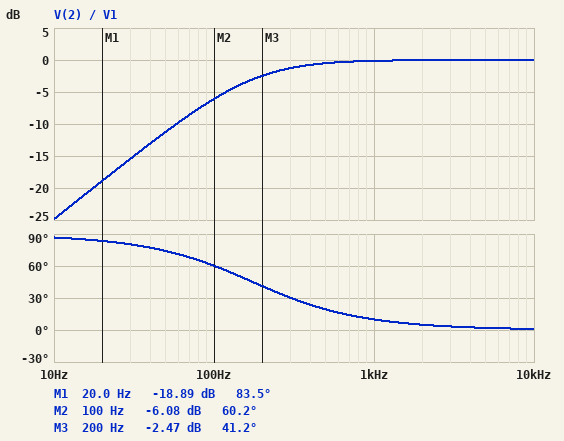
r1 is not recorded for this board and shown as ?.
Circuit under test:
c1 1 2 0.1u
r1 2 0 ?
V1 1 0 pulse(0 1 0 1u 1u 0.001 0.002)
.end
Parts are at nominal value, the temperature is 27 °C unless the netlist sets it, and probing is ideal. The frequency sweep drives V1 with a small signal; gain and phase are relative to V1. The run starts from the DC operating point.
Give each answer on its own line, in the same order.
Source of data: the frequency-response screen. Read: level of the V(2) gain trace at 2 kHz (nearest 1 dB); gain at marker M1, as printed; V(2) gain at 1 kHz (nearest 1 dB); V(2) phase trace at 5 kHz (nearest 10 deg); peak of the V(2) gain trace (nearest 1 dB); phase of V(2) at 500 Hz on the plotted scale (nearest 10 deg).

0 dB
-18.89 dB
0 dB
0 deg
0 dB
20 deg
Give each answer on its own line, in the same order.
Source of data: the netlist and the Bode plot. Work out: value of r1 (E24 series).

9.1 kΩ
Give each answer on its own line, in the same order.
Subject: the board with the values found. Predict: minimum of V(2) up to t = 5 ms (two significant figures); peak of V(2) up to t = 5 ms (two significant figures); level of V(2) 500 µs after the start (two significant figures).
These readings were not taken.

-740 mV
1.0 V
580 mV
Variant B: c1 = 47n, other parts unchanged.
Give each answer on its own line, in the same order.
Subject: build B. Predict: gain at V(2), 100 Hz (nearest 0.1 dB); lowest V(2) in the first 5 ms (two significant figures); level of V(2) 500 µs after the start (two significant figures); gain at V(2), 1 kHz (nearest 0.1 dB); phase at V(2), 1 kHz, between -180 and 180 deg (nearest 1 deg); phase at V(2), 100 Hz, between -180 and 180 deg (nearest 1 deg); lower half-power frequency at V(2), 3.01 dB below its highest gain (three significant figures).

-11.7 dB
-910 mV
310 mV
-0.6 dB
20 deg
75 deg
372 Hz
